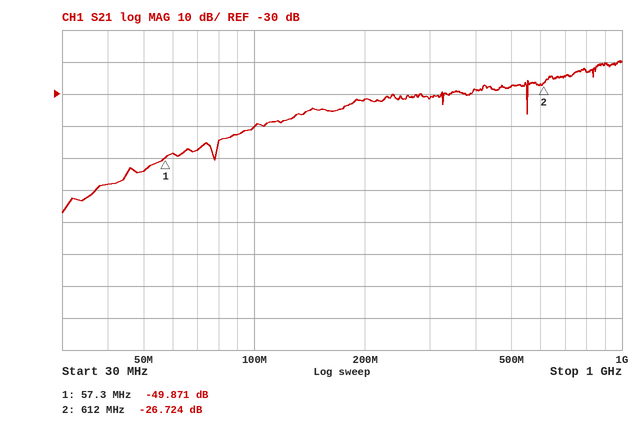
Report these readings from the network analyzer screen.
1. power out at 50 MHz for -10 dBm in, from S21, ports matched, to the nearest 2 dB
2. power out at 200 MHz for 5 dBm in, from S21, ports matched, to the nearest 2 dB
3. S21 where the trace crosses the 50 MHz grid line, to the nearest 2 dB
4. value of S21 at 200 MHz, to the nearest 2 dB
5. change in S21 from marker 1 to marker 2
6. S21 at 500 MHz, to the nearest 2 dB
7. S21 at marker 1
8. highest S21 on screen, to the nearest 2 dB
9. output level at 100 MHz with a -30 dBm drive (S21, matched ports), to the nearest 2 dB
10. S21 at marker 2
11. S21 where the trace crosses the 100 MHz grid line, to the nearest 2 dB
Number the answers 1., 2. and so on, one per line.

1. -64 dBm
2. -26 dBm
3. -54 dB
4. -32 dB
5. 23.147 dB
6. -28 dB
7. -49.871 dB
8. -20 dB
9. -70 dBm
10. -26.724 dB
11. -40 dB
